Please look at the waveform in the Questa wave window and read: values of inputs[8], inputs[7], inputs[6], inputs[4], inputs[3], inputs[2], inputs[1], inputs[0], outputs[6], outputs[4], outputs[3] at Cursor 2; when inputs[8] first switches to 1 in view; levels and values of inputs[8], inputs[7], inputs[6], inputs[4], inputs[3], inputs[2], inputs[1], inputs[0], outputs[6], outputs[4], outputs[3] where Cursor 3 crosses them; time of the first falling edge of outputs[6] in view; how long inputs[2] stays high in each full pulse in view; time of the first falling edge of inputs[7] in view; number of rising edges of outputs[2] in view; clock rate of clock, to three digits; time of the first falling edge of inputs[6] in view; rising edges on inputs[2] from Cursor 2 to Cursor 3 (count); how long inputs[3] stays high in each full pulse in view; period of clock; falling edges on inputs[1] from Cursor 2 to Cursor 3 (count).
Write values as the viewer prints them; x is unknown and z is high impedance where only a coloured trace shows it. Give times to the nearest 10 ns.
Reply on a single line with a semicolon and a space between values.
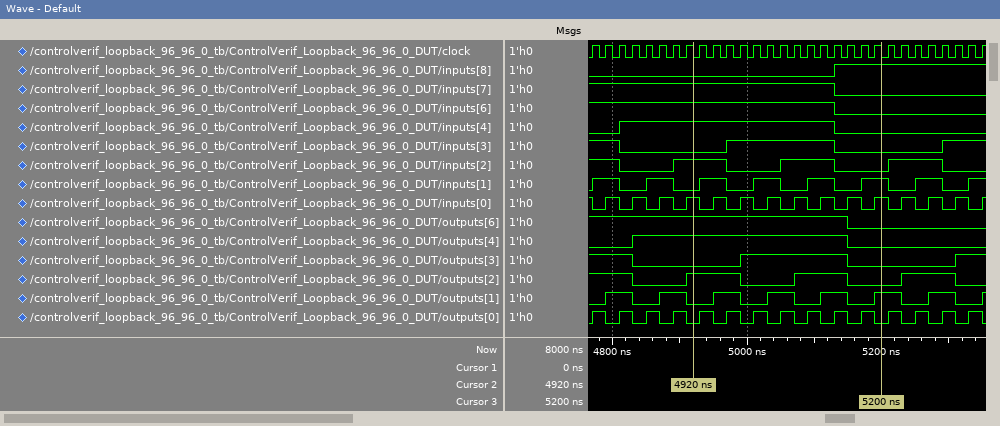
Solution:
inputs[8]=0, inputs[7]=1, inputs[6]=1, inputs[4]=1, inputs[3]=0, inputs[2]=1, inputs[1]=0, inputs[0]=1, outputs[6]=1, outputs[4]=1, outputs[3]=0; 5130 ns; inputs[8]=1, inputs[7]=0, inputs[6]=0, inputs[4]=0, inputs[3]=0, inputs[2]=0, inputs[1]=1, inputs[0]=1, outputs[6]=0, outputs[4]=0, outputs[3]=0; 5150 ns; 80 ns, 80 ns, 80 ns; 5130 ns; 3; 50.0 MHz; 5130 ns; 1; 160 ns; 20 ns; 3
